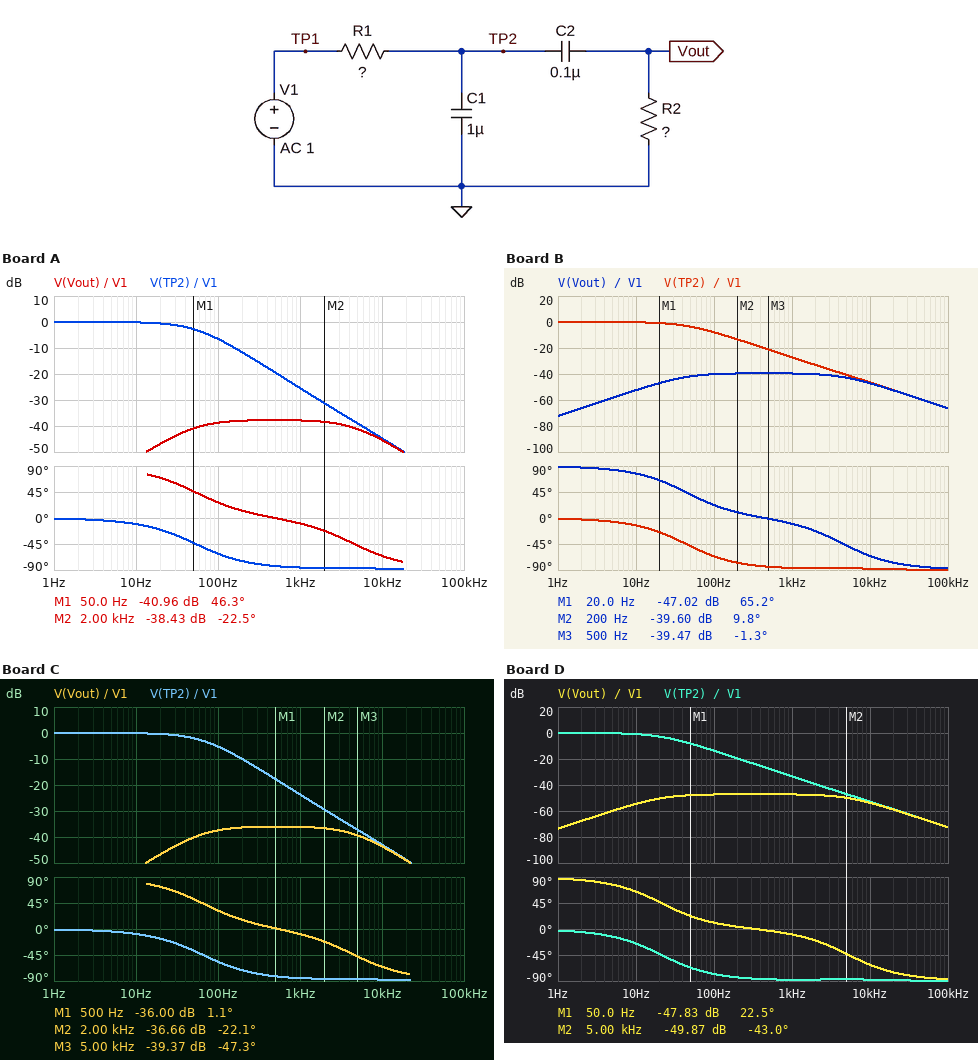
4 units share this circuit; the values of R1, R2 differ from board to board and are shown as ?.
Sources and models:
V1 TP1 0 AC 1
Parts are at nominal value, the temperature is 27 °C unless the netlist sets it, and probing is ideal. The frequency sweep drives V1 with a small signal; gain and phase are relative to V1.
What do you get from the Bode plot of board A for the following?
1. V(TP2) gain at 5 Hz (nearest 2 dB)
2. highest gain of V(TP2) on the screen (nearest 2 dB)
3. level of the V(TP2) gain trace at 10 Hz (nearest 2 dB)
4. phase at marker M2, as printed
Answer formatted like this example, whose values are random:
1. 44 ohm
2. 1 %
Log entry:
1. 0 dB
2. 0 dB
3. 0 dB
4. -22.5 deg
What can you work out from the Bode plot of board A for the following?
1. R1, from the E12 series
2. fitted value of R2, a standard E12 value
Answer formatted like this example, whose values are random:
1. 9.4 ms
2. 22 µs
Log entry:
1. 2.7 kΩ
2. 390 Ω
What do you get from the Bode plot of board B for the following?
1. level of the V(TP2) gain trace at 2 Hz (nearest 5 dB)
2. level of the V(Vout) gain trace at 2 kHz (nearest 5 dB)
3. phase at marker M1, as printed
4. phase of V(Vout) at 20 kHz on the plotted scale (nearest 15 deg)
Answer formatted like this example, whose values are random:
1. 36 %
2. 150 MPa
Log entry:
1. 0 dB
2. -40 dB
3. 65.2 deg
4. -75 deg
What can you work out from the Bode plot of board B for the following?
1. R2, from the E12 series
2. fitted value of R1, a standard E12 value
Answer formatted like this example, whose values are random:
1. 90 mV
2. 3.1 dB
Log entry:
1. 390 Ω
2. 3.3 kΩ
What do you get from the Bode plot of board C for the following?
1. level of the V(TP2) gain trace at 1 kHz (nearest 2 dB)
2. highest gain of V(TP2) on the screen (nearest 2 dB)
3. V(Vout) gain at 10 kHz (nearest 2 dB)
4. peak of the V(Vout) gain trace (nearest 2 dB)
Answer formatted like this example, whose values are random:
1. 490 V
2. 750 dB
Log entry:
1. -24 dB
2. 0 dB
3. -44 dB
4. -36 dB
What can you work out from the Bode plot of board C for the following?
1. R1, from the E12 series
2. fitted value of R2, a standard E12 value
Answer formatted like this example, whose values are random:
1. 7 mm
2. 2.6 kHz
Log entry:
1. 2.2 kΩ
2. 390 Ω
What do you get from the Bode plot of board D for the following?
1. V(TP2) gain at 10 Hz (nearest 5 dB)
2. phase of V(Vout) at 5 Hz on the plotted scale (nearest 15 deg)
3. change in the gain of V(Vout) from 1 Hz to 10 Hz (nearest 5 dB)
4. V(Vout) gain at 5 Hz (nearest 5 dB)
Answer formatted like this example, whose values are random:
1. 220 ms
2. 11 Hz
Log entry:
1. 0 dB
2. 75 deg
3. 20 dB
4. -60 dB
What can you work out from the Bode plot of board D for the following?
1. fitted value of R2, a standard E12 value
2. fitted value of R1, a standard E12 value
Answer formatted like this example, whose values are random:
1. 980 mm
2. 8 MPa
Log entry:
1. 330 Ω
2. 6.8 kΩ
